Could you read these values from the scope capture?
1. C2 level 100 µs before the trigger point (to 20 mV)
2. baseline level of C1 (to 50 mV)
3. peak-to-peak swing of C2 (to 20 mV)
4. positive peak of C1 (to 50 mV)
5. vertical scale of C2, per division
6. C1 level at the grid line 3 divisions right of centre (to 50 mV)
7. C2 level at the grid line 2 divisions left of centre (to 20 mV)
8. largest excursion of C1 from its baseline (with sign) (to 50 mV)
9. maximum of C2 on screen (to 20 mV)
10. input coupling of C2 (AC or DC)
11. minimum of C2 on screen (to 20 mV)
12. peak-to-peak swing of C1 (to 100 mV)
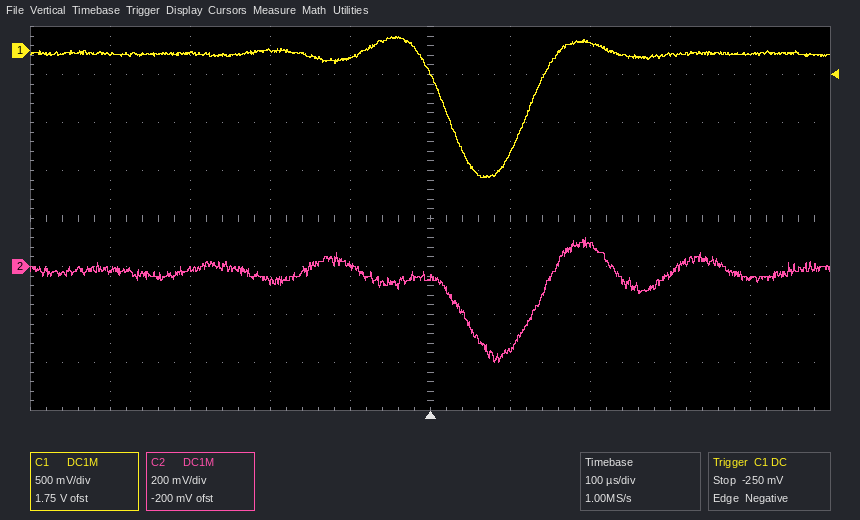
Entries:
0 mV
-50 mV
520 mV
150 mV
200 mV
-50 mV
-60 mV
-1.30 V
120 mV
DC
-400 mV
1.50 V
